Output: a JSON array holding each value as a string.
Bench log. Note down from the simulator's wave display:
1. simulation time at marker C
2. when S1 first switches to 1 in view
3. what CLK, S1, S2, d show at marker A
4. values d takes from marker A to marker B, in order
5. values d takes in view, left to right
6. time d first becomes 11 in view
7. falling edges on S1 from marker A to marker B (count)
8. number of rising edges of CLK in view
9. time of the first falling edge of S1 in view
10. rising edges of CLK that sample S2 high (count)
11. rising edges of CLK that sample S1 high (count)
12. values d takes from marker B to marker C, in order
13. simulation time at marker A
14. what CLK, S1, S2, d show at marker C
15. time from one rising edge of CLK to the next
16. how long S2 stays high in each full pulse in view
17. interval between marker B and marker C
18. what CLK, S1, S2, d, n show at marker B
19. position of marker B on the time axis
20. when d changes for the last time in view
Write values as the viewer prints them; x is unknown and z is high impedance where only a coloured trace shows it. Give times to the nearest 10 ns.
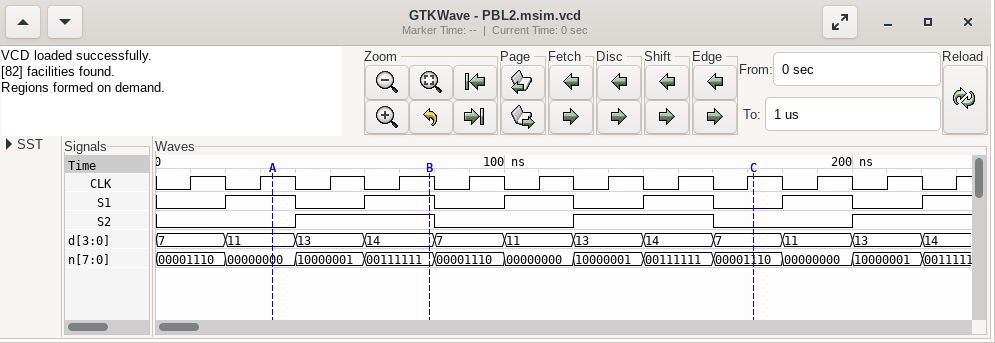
["170 ns", "20 ns", "CLK=1, S1=1, S2=0, d=11", "11, 13, 14", "7, 11, 13, 14, 7, 11, 13, 14, 7, 11, 13, 14", "20 ns", "1", "12", "40 ns", "6", "6", "14, 7, 11, 13, 14, 7", "30 ns", "CLK=1, S1=0, S2=0, d=7", "20 ns", "40 ns, 40 ns", "90 ns", "CLK=1, S1=1, S2=1, d=14, n=00111111", "80 ns", "220 ns"]
